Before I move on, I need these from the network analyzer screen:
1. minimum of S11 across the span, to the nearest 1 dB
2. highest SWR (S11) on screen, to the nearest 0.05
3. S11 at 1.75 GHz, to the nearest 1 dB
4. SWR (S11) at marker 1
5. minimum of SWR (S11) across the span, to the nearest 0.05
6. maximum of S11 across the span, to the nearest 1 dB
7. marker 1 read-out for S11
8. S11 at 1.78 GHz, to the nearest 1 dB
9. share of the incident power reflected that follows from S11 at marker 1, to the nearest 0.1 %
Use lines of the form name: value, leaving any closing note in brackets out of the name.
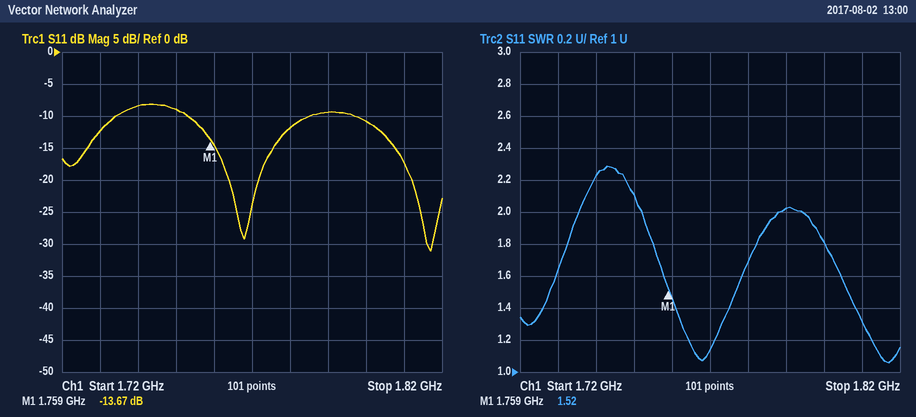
minimum of S11 across the span, to the nearest 1 dB: -31 dB
highest SWR (S11) on screen, to the nearest 0.05: 2.30
S11 at 1.75 GHz, to the nearest 1 dB: -9 dB
SWR (S11) at marker 1: 1.52
minimum of SWR (S11) across the span, to the nearest 0.05: 1.05
maximum of S11 across the span, to the nearest 1 dB: -8 dB
marker 1 read-out for S11: -13.67 dB
S11 at 1.78 GHz, to the nearest 1 dB: -12 dB
share of the incident power reflected that follows from S11 at marker 1, to the nearest 0.1 %: 4.3 %
